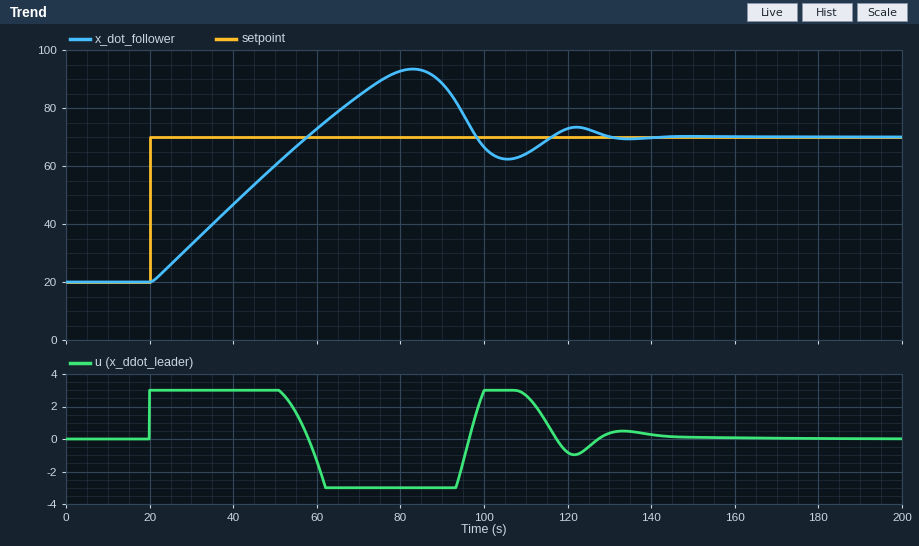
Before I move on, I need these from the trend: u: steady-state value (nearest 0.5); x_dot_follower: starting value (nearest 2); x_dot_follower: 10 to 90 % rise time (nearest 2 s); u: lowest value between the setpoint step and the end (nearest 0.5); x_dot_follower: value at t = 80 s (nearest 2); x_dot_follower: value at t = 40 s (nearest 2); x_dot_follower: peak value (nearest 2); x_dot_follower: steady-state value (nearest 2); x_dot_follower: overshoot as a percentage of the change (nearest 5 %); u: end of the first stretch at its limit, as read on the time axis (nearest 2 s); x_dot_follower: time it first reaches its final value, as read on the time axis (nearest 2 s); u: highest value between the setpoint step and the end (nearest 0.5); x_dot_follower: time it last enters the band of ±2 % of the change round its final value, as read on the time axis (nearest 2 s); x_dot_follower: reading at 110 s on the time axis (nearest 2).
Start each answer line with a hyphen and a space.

- 0.0
- 20
- 30 s
- -3.0
- 92
- 46
- 94
- 70
- 45 %
- 52 s
- 58 s
- 3.0
- 128 s
- 64
